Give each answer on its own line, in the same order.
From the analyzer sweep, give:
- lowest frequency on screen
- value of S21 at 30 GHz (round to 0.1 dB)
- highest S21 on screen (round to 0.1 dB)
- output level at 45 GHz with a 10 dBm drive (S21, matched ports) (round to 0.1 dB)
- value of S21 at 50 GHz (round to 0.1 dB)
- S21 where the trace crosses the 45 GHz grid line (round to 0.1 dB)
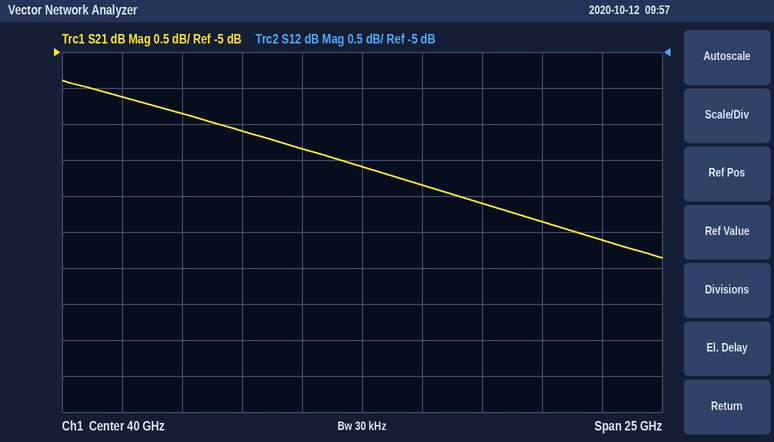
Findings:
27.5 GHz
-5.6 dB
-5.4 dB
2.9 dBm
-7.6 dB
-7.1 dB
